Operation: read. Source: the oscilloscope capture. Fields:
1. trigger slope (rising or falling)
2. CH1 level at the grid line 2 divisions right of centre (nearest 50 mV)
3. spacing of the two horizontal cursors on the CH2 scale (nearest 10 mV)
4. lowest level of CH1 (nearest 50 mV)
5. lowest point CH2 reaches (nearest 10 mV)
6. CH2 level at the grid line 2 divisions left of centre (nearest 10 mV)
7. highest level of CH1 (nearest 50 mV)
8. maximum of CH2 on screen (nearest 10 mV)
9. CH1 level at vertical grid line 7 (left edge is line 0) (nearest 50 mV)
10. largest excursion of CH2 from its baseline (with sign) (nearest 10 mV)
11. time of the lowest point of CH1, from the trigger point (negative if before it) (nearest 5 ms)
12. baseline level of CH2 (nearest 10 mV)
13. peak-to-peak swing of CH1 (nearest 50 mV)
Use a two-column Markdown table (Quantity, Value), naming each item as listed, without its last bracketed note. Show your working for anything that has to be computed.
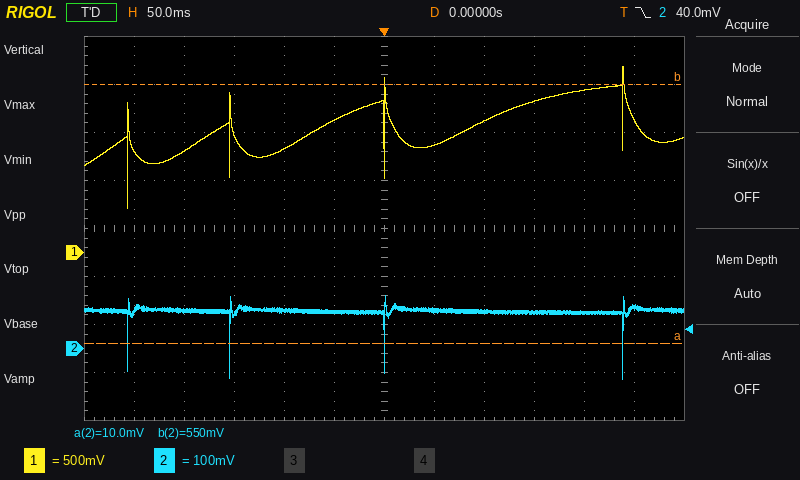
| Quantity | Value |
|---|---|
| trigger slope | falling |
| CH1 level at the grid line 2 divisions right of centre | 1.35 V |
| spacing of the two horizontal cursors on the CH2 scale | 540 mV |
| lowest level of CH1 | 450 mV |
| lowest point CH2 reaches | -60 mV |
| CH2 level at the grid line 2 divisions left of centre | 80 mV |
| highest level of CH1 | 1.95 V |
| maximum of CH2 on screen | 110 mV |
| CH1 level at vertical grid line 7 (left edge is line 0) | 1.10 V |
| largest excursion of CH2 from its baseline (with sign) | -60 mV − (80 mV) = -140 mV |
| time of the lowest point of CH1, from the trigger point (negative if before it) | -255 ms |
| baseline level of CH2 | 80 mV |
| peak-to-peak swing of CH1 | 1.95 V − (450 mV) = 1.50 V |
